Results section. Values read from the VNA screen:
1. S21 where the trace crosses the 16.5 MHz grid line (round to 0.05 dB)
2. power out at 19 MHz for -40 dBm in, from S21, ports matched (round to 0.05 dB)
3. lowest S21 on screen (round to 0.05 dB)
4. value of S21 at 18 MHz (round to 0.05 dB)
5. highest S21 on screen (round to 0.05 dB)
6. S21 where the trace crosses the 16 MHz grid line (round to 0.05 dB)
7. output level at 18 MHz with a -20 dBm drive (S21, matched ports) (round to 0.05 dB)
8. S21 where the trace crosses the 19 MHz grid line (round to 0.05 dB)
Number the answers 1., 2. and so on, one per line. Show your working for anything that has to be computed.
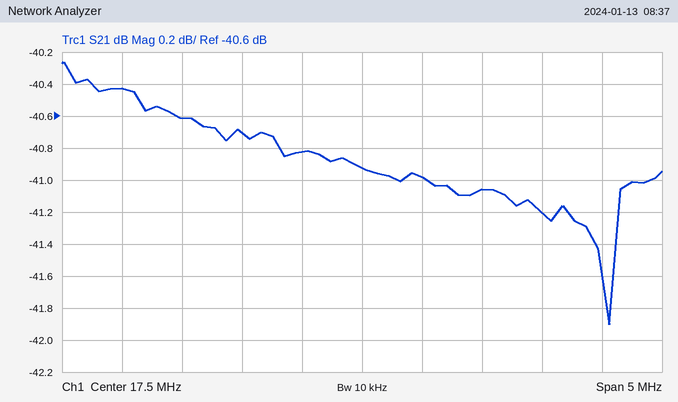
1. -40.70 dB
2. -40 dBm + (-41.20 dB) = -81.20 dBm
3. -41.90 dB
4. -41.00 dB
5. -40.25 dB
6. -40.60 dB
7. -20 dBm + (-41.00 dB) = -61.00 dBm
8. -41.20 dB
